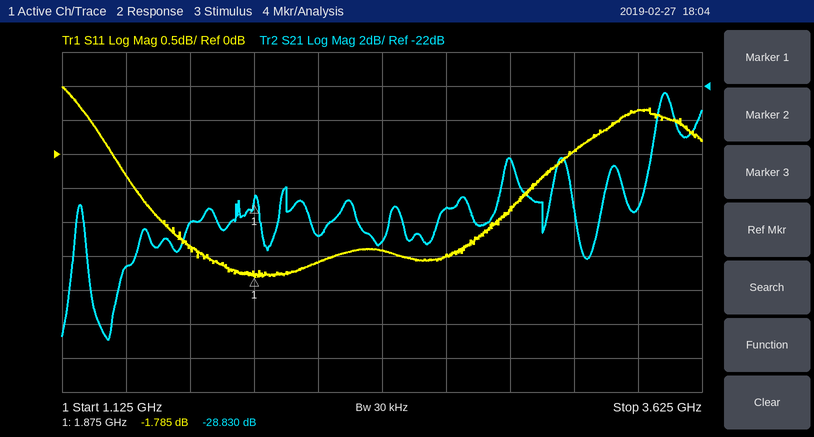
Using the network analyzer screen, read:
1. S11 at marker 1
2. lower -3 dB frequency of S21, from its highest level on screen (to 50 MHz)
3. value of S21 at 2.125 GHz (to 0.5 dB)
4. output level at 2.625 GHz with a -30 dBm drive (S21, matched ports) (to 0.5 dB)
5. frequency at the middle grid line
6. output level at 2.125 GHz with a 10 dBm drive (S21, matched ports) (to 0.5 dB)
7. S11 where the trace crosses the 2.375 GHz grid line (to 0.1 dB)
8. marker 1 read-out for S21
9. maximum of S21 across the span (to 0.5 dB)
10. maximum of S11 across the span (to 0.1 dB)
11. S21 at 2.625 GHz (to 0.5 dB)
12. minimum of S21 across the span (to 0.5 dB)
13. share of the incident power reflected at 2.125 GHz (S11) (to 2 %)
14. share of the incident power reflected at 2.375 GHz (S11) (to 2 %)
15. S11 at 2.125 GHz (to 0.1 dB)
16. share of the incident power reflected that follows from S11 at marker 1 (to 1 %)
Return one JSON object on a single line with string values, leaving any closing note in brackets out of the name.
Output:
{"S11 at marker 1": "-1.785 dB", "lower -3 dB frequency of S21, from its highest level on screen": "3.45 GHz", "value of S21 at 2.125 GHz": "-31.0 dB", "output level at 2.625 GHz with a -30 dBm drive (S21, matched ports)": "-59.0 dBm", "frequency at the middle grid line": "2.375 GHz", "output level at 2.125 GHz with a 10 dBm drive (S21, matched ports)": "-21.0 dBm", "S11 where the trace crosses the 2.375 GHz grid line": "-1.4 dB", "marker 1 read-out for S21": "-28.830 dB", "maximum of S21 across the span": "-22.5 dB", "maximum of S11 across the span": "1.0 dB", "S21 at 2.625 GHz": "-29.0 dB", "minimum of S21 across the span": "-37.0 dB", "share of the incident power reflected at 2.125 GHz (S11)": "70 %", "share of the incident power reflected at 2.375 GHz (S11)": "72 %", "S11 at 2.125 GHz": "-1.6 dB", "share of the incident power reflected that follows from S11 at marker 1": "66 %"}
